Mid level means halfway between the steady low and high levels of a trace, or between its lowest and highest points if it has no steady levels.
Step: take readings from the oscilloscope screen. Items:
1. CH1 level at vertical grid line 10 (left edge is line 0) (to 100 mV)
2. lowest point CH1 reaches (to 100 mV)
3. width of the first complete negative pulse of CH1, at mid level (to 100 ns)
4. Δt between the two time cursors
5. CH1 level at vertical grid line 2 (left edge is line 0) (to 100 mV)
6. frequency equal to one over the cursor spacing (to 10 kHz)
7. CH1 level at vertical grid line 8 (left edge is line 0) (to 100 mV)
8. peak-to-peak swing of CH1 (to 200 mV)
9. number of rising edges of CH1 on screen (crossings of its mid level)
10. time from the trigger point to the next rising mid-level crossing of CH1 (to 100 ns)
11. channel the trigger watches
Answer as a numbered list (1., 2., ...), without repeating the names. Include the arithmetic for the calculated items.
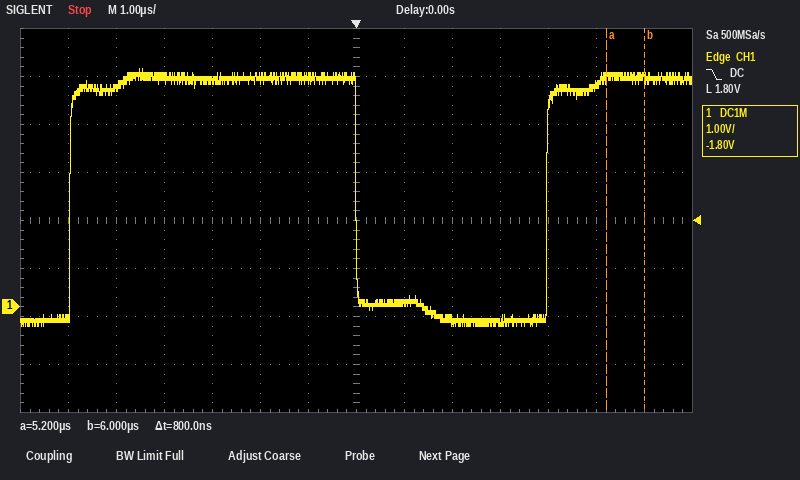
1. -300 mV
2. -400 mV
3. 4.0 µs
4. 800 ns
5. 4.6 V
6. 1 / 800 ns ≈ 1.25 MHz
7. 100 mV
8. 5.4 V
9. 2
10. 4.0 µs
11. CH1
